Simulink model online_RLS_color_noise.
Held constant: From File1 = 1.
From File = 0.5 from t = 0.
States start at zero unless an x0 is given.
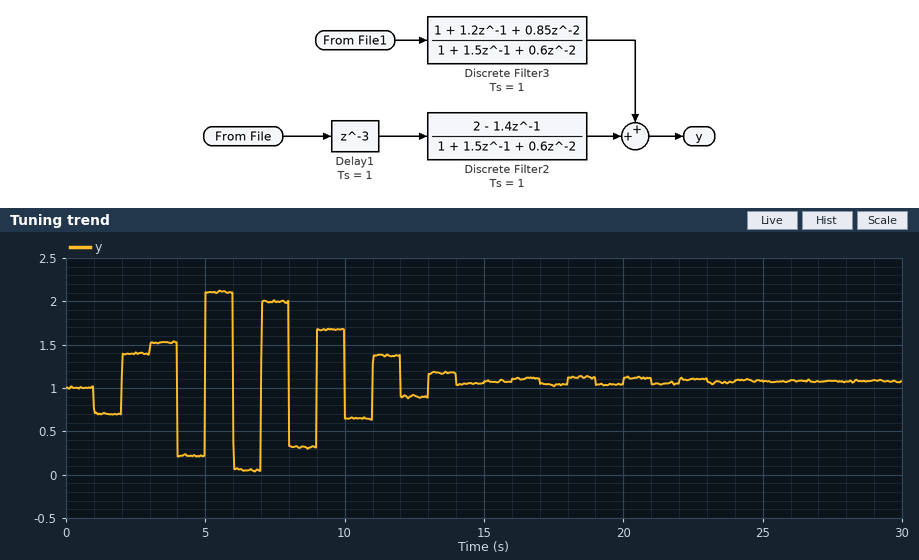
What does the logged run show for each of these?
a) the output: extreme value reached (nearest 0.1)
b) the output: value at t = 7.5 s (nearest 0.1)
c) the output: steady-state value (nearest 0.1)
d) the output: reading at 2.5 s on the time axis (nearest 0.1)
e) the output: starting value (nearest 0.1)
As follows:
2.1
2.0
1.1
1.4
1.0
